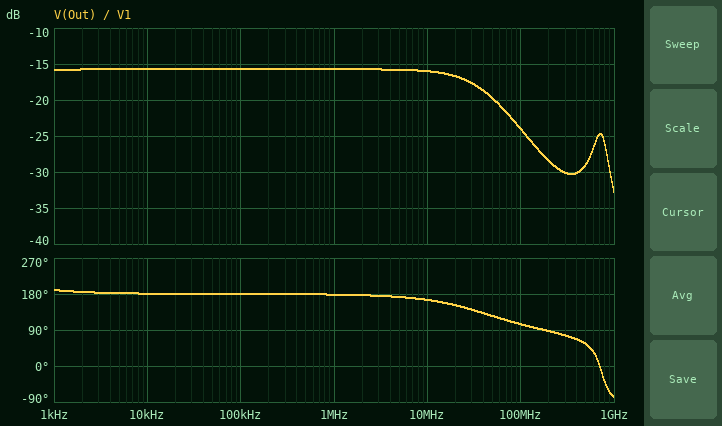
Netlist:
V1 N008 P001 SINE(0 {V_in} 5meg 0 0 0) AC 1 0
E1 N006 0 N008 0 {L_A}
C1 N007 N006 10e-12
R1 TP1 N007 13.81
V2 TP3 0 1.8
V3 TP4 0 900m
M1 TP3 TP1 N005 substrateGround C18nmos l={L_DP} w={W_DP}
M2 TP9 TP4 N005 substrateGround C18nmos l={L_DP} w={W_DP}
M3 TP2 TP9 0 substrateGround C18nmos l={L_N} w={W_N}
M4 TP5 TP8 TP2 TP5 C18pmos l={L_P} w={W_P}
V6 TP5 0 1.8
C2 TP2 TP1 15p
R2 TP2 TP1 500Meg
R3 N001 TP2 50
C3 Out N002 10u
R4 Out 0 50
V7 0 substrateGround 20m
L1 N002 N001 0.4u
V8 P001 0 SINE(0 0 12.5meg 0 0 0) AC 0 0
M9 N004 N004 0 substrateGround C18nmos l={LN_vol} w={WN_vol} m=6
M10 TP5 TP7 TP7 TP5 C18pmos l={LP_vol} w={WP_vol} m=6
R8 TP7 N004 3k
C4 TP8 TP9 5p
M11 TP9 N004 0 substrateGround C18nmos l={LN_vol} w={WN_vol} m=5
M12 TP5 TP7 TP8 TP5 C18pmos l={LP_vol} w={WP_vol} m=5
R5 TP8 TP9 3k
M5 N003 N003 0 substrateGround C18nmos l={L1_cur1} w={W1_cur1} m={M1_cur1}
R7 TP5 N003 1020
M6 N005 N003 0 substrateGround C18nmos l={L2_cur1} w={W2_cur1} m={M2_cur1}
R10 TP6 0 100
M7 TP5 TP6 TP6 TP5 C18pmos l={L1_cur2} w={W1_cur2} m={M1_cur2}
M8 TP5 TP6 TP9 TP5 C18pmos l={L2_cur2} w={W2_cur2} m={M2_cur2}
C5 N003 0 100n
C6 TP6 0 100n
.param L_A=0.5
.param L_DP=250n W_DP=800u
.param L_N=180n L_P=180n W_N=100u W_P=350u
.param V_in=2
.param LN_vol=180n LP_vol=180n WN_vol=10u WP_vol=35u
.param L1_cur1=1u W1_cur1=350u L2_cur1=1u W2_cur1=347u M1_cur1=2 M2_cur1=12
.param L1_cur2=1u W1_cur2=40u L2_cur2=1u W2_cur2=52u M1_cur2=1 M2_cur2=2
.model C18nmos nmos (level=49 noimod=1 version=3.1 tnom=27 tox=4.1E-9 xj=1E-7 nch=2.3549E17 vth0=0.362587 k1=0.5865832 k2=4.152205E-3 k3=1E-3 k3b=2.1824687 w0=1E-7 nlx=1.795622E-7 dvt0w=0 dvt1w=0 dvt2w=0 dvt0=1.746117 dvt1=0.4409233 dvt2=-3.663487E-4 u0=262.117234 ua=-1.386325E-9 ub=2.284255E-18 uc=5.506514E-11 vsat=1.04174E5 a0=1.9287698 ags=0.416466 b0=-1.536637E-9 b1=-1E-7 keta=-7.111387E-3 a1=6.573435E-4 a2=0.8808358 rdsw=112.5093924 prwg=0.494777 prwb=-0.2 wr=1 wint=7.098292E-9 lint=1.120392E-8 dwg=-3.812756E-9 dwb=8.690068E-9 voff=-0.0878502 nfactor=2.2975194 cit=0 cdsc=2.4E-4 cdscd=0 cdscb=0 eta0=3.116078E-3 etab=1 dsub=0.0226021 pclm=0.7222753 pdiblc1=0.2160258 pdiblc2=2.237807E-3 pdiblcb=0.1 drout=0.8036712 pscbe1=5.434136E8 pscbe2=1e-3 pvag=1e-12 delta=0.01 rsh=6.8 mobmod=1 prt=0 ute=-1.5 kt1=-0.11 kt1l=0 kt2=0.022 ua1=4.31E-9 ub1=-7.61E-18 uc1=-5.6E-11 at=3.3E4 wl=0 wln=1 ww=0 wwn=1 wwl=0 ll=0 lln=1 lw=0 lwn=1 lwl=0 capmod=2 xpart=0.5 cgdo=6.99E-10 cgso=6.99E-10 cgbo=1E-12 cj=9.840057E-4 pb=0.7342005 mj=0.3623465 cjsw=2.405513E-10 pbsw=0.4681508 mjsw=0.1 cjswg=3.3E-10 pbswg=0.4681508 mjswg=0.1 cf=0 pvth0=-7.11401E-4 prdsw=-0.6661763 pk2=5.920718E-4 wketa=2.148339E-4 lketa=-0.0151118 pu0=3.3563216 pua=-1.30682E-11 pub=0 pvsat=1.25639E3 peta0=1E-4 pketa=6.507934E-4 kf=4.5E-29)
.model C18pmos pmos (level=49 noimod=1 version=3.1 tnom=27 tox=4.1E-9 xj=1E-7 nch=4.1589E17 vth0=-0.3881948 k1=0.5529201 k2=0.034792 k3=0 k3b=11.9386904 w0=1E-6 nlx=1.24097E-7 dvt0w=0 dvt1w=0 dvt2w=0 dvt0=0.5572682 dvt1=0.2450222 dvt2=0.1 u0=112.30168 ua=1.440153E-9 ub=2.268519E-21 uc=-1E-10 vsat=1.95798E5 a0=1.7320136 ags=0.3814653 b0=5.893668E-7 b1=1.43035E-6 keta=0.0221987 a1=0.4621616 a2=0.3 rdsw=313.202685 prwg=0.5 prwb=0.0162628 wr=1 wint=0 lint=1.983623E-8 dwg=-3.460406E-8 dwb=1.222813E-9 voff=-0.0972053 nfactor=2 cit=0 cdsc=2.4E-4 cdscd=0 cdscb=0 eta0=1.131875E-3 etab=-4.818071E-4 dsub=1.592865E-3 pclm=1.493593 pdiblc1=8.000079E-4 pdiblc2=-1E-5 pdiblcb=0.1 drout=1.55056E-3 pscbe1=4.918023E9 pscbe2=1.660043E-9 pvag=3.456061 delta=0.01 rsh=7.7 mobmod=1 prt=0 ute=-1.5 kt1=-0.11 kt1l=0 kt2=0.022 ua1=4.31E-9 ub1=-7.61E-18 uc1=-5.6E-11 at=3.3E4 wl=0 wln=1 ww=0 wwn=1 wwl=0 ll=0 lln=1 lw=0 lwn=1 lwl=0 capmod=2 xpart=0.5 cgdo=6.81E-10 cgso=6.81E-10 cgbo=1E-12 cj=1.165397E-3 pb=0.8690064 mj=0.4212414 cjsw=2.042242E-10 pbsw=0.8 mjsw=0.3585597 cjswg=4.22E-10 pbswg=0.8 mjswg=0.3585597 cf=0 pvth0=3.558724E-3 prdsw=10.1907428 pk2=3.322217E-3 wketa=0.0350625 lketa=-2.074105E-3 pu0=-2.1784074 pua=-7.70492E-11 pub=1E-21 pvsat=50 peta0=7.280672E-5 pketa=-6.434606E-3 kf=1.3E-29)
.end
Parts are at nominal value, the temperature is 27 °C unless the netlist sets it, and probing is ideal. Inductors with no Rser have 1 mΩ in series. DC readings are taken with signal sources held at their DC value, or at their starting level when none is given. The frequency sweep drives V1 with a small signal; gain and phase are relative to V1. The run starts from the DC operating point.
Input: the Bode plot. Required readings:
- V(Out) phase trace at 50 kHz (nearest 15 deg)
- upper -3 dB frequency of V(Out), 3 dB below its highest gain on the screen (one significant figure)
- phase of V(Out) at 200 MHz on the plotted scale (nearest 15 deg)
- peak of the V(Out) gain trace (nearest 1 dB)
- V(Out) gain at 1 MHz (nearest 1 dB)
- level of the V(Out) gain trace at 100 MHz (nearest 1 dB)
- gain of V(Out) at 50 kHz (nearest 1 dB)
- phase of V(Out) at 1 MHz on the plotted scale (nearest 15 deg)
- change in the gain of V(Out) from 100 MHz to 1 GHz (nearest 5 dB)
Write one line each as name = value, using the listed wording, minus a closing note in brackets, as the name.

V(Out) phase trace at 50 kHz = 180 deg
upper -3 dB frequency of V(Out), 3 dB below its highest gain on the screen = 40 MHz
phase of V(Out) at 200 MHz on the plotted scale = 90 deg
peak of the V(Out) gain trace = -16 dB
V(Out) gain at 1 MHz = -16 dB
level of the V(Out) gain trace at 100 MHz = -24 dB
gain of V(Out) at 50 kHz = -16 dB
phase of V(Out) at 1 MHz on the plotted scale = 180 deg
change in the gain of V(Out) from 100 MHz to 1 GHz = -10 dB
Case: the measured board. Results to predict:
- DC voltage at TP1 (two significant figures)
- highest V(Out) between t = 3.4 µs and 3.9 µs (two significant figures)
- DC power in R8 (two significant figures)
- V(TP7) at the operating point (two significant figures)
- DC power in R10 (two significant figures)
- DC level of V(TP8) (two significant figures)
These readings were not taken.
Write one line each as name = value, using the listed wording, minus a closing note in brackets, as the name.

DC voltage at TP1 = 890 mV
highest V(Out) between t = 3.4 µs and 3.9 µs = 290 mV
DC power in R8 = 170 µW
V(TP7) at the operating point = 1.3 V
DC power in R10 = 190 µW
DC level of V(TP8) = 1.2 V
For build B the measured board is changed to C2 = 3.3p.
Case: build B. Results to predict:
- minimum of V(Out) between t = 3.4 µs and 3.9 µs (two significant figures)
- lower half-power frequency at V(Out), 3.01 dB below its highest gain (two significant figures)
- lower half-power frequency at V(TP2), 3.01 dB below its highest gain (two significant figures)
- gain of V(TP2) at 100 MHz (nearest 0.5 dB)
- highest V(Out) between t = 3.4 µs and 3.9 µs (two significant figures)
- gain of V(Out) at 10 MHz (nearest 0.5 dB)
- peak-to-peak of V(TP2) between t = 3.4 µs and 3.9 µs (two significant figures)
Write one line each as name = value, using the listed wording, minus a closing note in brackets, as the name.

minimum of V(Out) between t = 3.4 µs and 3.9 µs = -370 mV
lower half-power frequency at V(Out), 3.01 dB below its highest gain = 190 Hz
lower half-power frequency at V(TP2), 3.01 dB below its highest gain = 470 MHz
gain of V(TP2) at 100 MHz = 3.5 dB
highest V(Out) between t = 3.4 µs and 3.9 µs = 340 mV
gain of V(Out) at 10 MHz = -3.0 dB
peak-to-peak of V(TP2) between t = 3.4 µs and 3.9 µs = 1.5 V
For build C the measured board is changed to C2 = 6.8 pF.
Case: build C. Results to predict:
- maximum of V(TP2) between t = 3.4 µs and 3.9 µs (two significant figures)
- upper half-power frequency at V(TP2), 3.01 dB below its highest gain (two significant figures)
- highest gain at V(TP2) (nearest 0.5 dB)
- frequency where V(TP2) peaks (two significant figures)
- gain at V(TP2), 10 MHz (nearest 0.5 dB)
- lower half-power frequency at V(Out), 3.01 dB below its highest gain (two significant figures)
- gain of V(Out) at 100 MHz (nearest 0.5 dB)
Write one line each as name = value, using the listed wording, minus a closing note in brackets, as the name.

maximum of V(TP2) between t = 3.4 µs and 3.9 µs = 1.6 V
upper half-power frequency at V(TP2), 3.01 dB below its highest gain = 880 MHz
highest gain at V(TP2) = 8.5 dB
frequency where V(TP2) peaks = 720 MHz
gain at V(TP2), 10 MHz = -3.0 dB
lower half-power frequency at V(Out), 3.01 dB below its highest gain = 170 Hz
gain of V(Out) at 100 MHz = -17.5 dB
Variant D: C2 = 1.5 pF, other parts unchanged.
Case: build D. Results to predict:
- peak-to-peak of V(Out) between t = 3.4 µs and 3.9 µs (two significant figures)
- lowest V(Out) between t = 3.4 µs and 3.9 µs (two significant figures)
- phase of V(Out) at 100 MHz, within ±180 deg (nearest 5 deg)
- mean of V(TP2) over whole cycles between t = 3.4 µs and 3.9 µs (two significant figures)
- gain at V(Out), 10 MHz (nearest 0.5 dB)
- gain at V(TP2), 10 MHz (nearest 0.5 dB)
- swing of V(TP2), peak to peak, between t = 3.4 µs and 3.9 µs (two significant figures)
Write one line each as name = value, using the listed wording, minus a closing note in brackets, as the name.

peak-to-peak of V(Out) between t = 3.4 µs and 3.9 µs = 710 mV
lowest V(Out) between t = 3.4 µs and 3.9 µs = -370 mV
phase of V(Out) at 100 MHz, within ±180 deg = 100 deg
mean of V(TP2) over whole cycles between t = 3.4 µs and 3.9 µs = 870 mV
gain at V(Out), 10 MHz = 3.5 dB
gain at V(TP2), 10 MHz = 9.5 dB
swing of V(TP2), peak to peak, between t = 3.4 µs and 3.9 µs = 1.6 V
